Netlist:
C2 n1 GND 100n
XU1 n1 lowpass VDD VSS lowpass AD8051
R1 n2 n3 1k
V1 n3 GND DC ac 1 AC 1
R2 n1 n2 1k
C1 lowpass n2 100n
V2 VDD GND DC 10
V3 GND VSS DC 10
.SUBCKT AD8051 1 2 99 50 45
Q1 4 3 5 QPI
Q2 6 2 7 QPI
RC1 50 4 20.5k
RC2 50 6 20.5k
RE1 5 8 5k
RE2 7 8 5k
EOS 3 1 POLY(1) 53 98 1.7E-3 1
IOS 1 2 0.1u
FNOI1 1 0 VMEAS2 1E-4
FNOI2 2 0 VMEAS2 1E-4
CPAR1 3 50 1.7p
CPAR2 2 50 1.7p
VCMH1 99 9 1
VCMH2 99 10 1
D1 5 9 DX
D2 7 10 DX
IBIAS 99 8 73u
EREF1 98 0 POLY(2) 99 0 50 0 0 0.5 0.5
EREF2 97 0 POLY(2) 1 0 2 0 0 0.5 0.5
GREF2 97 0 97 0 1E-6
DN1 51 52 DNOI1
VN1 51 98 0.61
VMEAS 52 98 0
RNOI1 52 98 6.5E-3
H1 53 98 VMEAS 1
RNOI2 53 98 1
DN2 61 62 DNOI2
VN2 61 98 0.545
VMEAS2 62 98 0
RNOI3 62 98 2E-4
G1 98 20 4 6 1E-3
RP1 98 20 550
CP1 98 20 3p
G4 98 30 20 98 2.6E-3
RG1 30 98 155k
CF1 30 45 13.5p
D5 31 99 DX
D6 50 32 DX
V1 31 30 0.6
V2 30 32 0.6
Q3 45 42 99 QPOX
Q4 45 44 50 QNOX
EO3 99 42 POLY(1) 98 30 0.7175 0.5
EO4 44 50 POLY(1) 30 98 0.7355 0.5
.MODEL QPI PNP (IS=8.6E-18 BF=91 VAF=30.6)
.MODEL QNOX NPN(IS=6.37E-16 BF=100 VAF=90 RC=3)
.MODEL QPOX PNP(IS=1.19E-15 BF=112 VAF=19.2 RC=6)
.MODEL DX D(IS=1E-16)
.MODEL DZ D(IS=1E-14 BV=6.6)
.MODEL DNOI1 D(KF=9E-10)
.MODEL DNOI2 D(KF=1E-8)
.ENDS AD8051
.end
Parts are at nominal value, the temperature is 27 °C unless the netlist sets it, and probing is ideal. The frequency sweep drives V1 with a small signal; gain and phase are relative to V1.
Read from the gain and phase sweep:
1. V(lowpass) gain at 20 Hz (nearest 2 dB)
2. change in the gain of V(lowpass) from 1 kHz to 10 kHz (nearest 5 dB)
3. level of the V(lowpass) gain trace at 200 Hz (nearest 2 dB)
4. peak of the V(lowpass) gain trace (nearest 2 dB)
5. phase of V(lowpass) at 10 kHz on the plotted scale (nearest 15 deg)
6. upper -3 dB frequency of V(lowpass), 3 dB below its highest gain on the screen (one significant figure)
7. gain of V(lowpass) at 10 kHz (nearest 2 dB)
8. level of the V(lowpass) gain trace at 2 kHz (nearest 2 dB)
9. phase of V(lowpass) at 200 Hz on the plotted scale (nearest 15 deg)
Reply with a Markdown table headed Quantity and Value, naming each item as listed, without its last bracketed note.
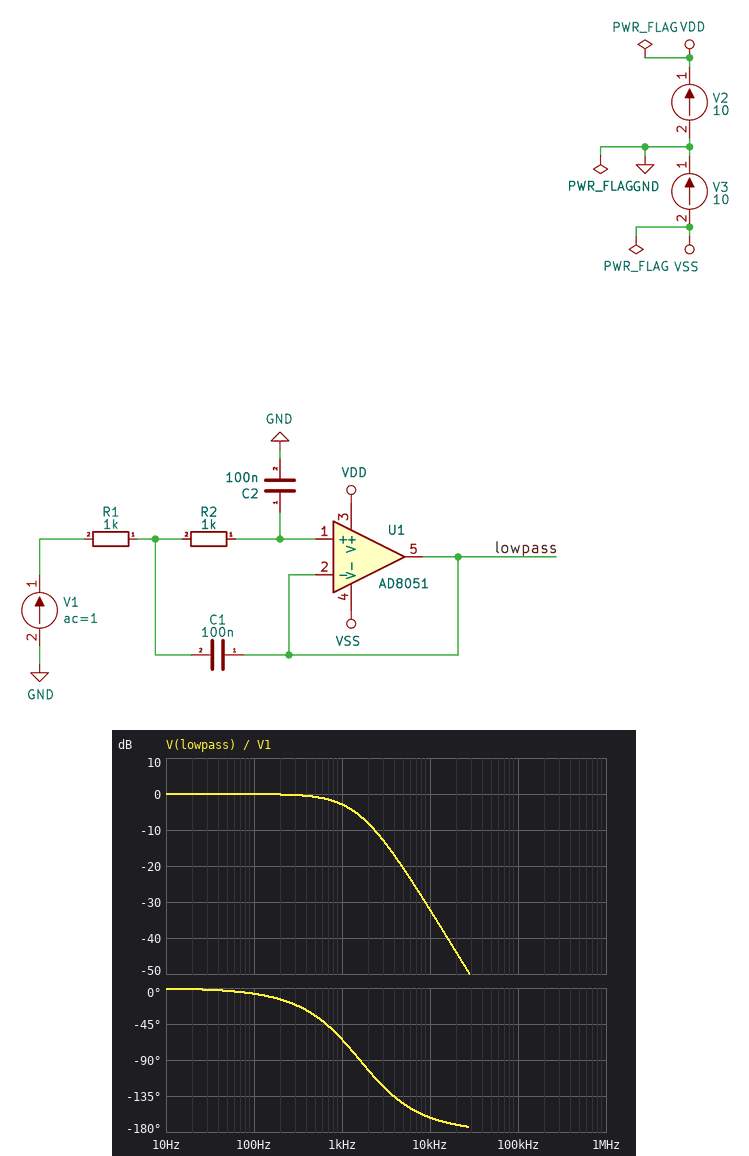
| Quantity | Value |
|---|---|
| V(lowpass) gain at 20 Hz | 0 dB |
| change in the gain of V(lowpass) from 1 kHz to 10 kHz | -30 dB |
| level of the V(lowpass) gain trace at 200 Hz | 0 dB |
| peak of the V(lowpass) gain trace | 0 dB |
| phase of V(lowpass) at 10 kHz on the plotted scale | -165 deg |
| upper -3 dB frequency of V(lowpass), 3 dB below its highest gain on the screen | 1 kHz |
| gain of V(lowpass) at 10 kHz | -32 dB |
| level of the V(lowpass) gain trace at 2 kHz | -8 dB |
| phase of V(lowpass) at 200 Hz on the plotted scale | -15 deg |
